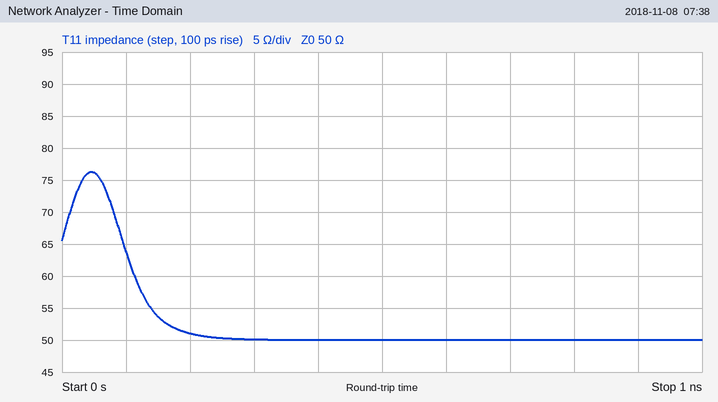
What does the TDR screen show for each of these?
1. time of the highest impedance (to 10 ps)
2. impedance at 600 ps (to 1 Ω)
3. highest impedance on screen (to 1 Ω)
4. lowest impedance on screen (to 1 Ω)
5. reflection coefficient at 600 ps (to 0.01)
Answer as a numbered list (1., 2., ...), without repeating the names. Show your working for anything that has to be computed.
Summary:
1. 50 ps
2. 50 Ω
3. 76 Ω
4. 50 Ω
5. (50 − 50)/(50 + 50) ≈ 0.00
